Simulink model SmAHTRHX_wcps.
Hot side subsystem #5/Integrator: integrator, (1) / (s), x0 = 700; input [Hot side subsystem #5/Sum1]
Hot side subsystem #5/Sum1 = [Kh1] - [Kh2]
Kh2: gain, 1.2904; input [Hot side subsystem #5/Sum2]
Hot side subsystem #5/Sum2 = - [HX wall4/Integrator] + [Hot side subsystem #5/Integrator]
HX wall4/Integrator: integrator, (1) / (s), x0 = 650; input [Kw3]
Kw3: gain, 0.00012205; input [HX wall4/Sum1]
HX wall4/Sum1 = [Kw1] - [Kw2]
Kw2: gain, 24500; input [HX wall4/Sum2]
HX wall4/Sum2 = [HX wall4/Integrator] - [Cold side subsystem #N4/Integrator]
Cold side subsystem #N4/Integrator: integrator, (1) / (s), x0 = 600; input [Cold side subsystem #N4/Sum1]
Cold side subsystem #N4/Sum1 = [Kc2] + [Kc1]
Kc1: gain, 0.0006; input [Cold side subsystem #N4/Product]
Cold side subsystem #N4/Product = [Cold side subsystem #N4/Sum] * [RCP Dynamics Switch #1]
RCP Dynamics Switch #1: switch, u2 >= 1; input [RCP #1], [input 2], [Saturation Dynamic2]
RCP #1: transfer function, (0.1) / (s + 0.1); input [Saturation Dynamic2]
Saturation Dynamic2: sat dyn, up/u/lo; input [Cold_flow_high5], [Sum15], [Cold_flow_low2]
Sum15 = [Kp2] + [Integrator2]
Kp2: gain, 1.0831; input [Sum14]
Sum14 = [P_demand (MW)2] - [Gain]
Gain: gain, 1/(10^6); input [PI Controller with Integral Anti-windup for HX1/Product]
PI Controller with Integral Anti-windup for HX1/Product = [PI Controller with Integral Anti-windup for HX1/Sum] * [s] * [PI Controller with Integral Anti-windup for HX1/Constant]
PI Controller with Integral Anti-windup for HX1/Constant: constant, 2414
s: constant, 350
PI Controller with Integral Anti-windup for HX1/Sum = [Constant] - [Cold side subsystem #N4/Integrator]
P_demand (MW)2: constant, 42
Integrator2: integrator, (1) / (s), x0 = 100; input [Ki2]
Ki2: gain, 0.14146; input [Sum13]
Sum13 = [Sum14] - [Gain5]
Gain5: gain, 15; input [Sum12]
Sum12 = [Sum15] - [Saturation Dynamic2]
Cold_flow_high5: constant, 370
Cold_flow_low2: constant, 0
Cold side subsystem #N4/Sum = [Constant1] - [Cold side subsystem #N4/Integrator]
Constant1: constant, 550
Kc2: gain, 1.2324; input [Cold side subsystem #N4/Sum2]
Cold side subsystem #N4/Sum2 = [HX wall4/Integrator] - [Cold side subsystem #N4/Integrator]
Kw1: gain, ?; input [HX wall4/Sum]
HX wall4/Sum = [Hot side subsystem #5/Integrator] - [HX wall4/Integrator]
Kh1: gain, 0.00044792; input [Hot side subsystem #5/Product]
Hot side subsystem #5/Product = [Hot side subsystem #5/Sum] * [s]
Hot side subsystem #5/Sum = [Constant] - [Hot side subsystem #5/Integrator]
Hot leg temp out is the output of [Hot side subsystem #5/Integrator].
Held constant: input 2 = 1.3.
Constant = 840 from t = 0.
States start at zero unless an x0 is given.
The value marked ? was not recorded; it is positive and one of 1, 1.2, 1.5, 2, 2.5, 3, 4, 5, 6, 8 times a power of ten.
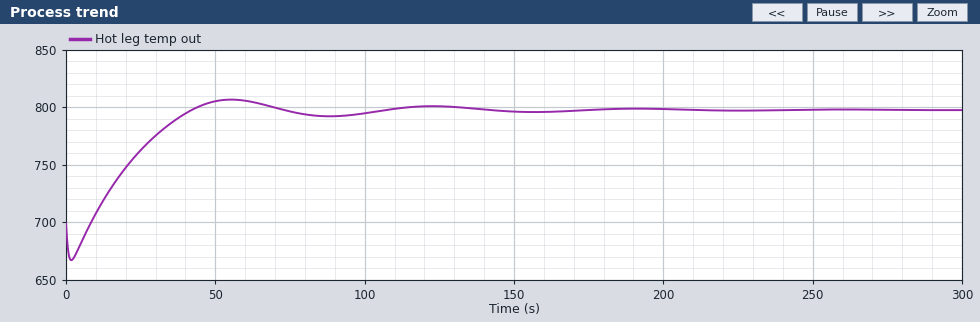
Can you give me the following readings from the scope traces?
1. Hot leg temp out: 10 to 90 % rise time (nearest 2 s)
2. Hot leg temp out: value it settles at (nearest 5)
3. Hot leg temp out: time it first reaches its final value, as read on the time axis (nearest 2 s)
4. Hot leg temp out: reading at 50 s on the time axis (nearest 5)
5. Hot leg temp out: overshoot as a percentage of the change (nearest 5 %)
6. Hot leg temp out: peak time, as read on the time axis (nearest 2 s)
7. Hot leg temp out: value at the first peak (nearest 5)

26 s
800
42 s
805
10 %
56 s
805
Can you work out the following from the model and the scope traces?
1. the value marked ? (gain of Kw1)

12000
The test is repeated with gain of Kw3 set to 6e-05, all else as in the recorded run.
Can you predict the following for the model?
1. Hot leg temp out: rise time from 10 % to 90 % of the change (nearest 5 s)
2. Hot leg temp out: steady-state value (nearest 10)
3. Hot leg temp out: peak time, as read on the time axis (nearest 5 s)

30 s
800
65 s
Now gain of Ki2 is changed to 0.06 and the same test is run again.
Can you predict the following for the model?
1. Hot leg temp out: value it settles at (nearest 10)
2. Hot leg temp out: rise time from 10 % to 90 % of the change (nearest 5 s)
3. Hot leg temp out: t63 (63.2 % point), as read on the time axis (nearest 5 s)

800
30 s
25 s
